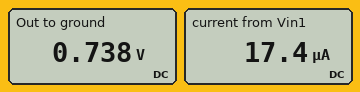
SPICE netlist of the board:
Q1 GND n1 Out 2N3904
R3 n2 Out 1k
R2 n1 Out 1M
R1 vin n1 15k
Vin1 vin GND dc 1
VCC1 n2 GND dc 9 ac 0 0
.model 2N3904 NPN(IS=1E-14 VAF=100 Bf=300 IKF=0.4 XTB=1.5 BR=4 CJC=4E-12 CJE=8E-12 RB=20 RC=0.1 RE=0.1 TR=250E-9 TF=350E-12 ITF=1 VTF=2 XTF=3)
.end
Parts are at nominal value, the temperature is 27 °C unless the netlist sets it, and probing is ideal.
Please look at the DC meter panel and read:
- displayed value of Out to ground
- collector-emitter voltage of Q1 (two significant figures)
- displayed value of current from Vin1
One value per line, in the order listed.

0.738 V
-740 mV
17.4 µA
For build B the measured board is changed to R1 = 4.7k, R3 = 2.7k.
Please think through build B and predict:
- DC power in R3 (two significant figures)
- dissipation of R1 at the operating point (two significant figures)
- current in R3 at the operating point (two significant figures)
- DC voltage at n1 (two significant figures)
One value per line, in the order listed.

26 mW
20 µW
3.1 mA
690 mV
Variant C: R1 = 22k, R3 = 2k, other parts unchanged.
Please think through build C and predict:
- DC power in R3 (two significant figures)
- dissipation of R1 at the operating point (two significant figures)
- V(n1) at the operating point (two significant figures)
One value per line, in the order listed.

34 mW
4.0 µW
700 mV
